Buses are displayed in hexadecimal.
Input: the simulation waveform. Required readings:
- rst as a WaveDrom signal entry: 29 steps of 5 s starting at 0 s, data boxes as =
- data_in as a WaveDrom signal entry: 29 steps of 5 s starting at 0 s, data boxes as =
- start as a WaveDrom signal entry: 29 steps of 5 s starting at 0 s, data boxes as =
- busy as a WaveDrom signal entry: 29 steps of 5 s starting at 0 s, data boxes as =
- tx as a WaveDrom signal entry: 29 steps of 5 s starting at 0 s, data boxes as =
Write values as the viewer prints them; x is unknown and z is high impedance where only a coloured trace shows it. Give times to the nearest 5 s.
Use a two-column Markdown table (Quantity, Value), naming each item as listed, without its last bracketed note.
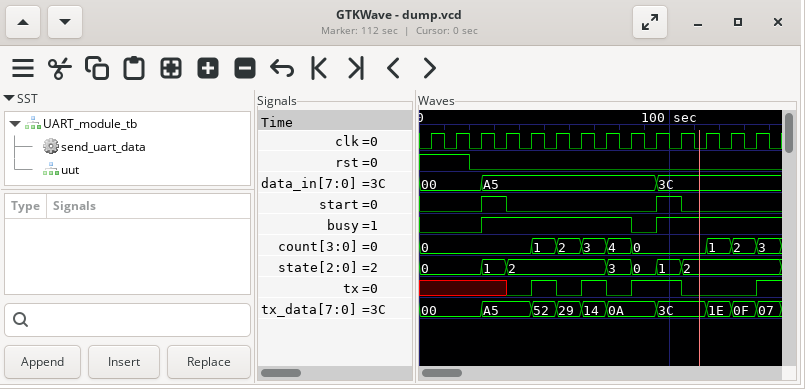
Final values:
| Quantity | Value |
|---|---|
| rst as a WaveDrom signal entry: 29 steps of 5 s starting at 0 s, data boxes as = | {name: 'rst', wave: '1...0........................'} |
| data_in as a WaveDrom signal entry: 29 steps of 5 s starting at 0 s, data boxes as = | {name: 'data_in', wave: '=....=.............=.........', data: '00 A5 3C'} |
| start as a WaveDrom signal entry: 29 steps of 5 s starting at 0 s, data boxes as = | {name: 'start', wave: '0....1.0...........1.0.......'} |
| busy as a WaveDrom signal entry: 29 steps of 5 s starting at 0 s, data boxes as = | {name: 'busy', wave: '0....1...........0.1.........'} |
| tx as a WaveDrom signal entry: 29 steps of 5 s starting at 0 s, data boxes as = | {name: 'tx', wave: 'x......0.1.0.1.0.1...0.....1.'} |
